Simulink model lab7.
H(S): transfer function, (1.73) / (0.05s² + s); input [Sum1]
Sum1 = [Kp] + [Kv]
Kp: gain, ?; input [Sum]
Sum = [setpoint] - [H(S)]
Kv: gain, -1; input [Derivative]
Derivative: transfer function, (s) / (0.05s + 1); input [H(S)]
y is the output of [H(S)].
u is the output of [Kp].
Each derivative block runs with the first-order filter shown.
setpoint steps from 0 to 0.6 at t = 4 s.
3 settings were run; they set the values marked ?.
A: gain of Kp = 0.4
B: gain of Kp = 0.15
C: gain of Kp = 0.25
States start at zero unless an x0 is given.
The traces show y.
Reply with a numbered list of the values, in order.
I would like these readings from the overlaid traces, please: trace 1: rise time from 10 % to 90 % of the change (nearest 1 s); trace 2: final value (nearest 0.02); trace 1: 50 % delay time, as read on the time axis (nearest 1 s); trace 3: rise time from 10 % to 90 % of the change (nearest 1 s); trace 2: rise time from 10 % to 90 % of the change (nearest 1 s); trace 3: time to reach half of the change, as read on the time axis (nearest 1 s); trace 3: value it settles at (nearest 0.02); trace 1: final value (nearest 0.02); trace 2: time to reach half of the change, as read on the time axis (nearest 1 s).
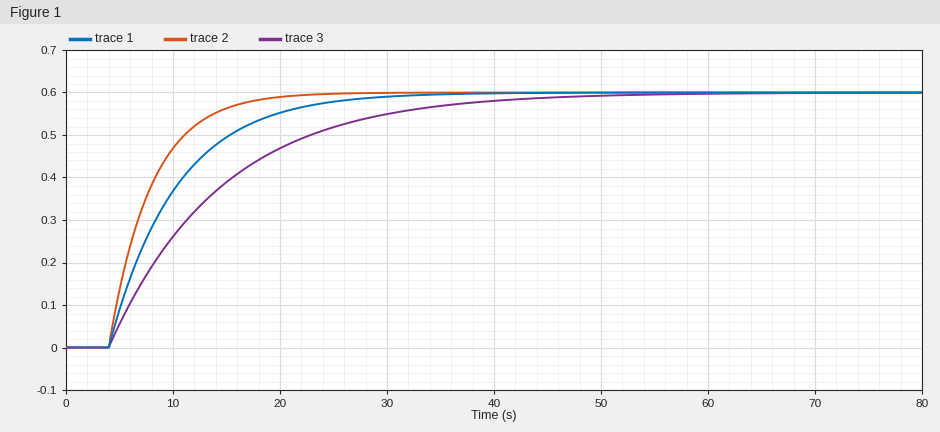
1. 14 s
2. 0.60
3. 8 s
4. 23 s
5. 9 s
6. 11 s
7. 0.60
8. 0.60
9. 7 s
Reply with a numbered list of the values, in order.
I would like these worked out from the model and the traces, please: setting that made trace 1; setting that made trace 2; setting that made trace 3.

1. C
2. A
3. B
